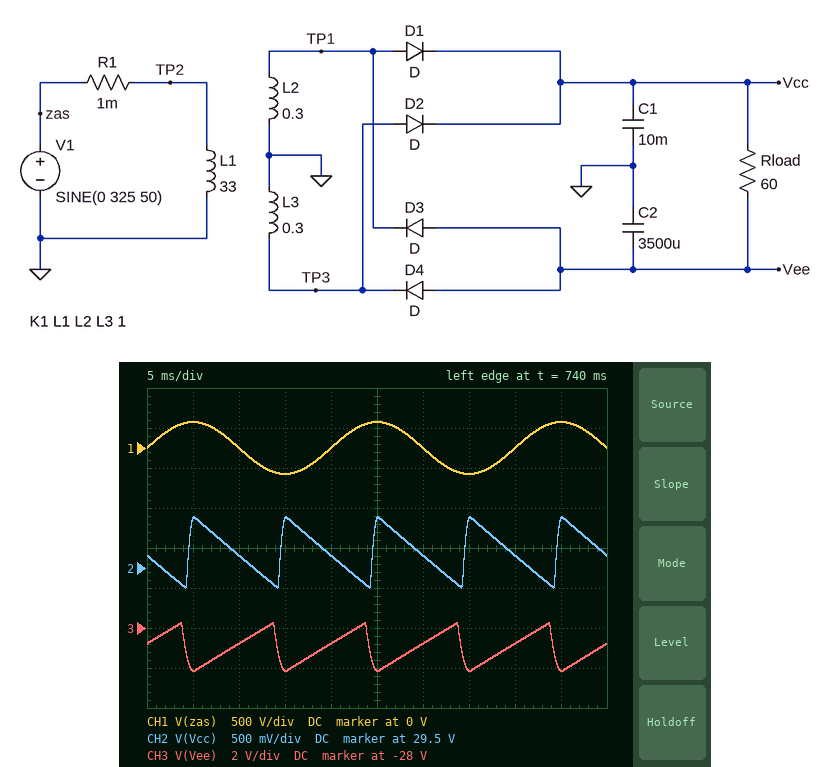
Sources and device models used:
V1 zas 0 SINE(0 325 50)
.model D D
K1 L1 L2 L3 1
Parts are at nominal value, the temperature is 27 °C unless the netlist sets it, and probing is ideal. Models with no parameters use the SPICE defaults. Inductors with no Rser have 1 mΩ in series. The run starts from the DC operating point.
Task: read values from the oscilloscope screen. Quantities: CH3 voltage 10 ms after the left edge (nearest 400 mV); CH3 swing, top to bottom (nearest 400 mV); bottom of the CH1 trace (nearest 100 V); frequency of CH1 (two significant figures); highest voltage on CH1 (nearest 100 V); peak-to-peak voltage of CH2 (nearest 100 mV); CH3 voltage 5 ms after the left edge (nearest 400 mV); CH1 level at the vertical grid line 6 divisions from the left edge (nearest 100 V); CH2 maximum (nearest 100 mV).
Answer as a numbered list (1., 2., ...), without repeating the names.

1. -28.8 V
2. 2.4 V
3. -300 V
4. 50 Hz
5. 300 V
6. 900 mV
7. -30.0 V
8. 0 V
9. 30.1 V
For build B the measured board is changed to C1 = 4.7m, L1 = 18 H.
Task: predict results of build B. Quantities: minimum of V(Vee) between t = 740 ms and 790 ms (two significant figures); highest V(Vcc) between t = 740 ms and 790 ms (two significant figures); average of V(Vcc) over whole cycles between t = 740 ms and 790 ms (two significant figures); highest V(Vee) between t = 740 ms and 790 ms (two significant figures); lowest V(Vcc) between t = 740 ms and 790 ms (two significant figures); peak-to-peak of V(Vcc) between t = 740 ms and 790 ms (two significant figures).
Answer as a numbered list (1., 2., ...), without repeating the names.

1. -41 V
2. 41 V
3. 40 V
4. -38 V
5. 39 V
6. 2.5 V
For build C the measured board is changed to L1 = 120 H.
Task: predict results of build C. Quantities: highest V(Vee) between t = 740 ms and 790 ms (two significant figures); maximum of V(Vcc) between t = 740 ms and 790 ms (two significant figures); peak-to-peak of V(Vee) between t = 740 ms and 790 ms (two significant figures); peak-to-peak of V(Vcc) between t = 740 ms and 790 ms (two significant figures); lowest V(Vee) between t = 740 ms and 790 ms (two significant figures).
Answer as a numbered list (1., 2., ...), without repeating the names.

1. -14 V
2. 15 V
3. 1.2 V
4. 450 mV
5. -15 V
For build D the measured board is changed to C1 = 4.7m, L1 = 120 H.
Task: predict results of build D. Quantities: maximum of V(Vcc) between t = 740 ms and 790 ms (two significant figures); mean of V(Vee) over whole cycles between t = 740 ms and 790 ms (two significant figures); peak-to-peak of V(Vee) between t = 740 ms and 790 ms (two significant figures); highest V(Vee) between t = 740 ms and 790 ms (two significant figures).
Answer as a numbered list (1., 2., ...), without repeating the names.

1. 15 V
2. -15 V
3. 1.2 V
4. -14 V
